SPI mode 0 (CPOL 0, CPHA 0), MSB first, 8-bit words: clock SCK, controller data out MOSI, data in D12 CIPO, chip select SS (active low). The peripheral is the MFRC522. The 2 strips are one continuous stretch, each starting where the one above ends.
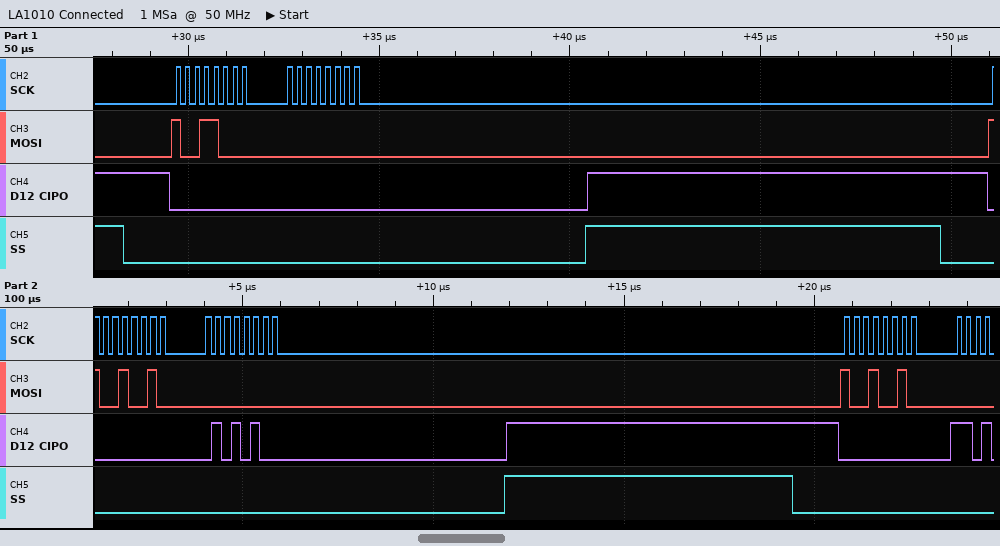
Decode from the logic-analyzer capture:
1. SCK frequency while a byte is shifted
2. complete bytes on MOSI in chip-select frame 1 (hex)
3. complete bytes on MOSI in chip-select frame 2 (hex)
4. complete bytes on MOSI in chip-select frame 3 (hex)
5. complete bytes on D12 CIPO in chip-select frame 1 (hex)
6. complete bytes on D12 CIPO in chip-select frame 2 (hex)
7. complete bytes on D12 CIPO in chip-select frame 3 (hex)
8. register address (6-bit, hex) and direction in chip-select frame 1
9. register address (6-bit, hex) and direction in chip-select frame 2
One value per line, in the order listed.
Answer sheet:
4 MHz
98 00
92 00
92
00 00
00 54
00
0x0C read
0x09 read
